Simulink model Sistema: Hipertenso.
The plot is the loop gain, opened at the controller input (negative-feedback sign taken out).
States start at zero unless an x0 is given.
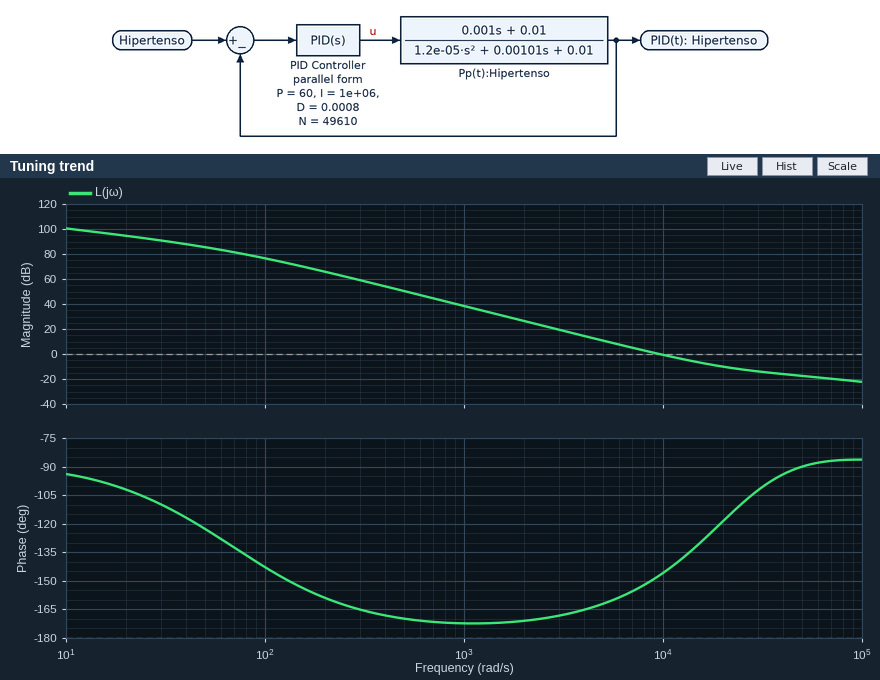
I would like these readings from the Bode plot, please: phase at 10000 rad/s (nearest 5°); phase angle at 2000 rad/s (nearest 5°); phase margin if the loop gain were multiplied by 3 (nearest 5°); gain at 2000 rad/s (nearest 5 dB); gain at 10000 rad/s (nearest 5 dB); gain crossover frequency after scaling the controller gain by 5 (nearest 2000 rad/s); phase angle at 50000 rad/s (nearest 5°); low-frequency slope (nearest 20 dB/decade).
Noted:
-145°
-170°
60°
25 dB
0 dB
30000 rad/s
-90°
-20 dB/decade
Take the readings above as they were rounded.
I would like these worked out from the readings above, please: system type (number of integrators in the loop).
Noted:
1
